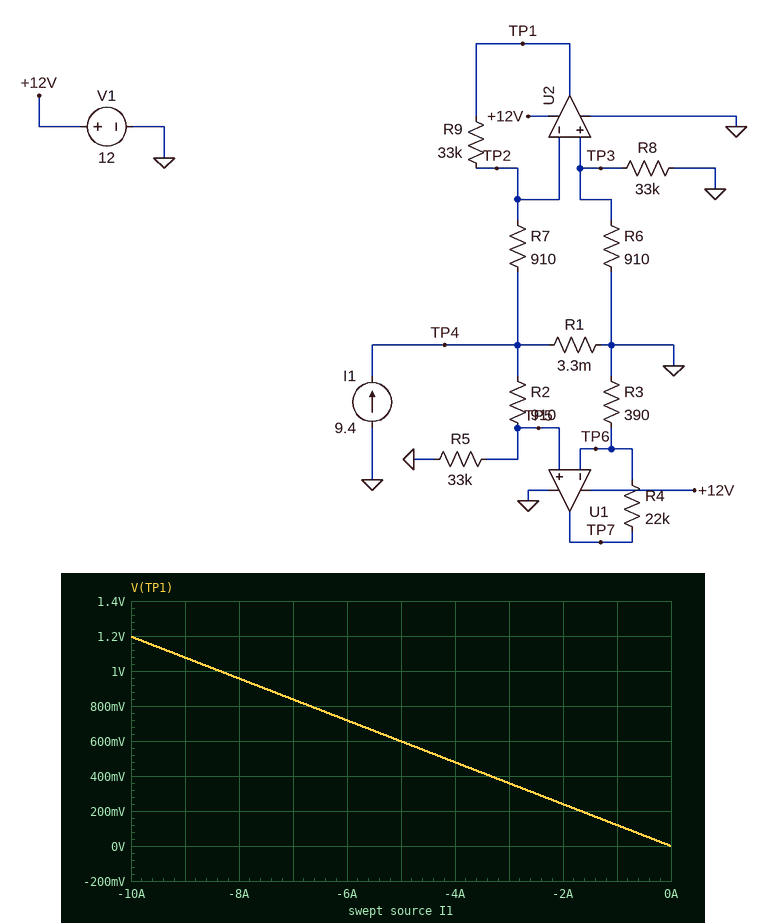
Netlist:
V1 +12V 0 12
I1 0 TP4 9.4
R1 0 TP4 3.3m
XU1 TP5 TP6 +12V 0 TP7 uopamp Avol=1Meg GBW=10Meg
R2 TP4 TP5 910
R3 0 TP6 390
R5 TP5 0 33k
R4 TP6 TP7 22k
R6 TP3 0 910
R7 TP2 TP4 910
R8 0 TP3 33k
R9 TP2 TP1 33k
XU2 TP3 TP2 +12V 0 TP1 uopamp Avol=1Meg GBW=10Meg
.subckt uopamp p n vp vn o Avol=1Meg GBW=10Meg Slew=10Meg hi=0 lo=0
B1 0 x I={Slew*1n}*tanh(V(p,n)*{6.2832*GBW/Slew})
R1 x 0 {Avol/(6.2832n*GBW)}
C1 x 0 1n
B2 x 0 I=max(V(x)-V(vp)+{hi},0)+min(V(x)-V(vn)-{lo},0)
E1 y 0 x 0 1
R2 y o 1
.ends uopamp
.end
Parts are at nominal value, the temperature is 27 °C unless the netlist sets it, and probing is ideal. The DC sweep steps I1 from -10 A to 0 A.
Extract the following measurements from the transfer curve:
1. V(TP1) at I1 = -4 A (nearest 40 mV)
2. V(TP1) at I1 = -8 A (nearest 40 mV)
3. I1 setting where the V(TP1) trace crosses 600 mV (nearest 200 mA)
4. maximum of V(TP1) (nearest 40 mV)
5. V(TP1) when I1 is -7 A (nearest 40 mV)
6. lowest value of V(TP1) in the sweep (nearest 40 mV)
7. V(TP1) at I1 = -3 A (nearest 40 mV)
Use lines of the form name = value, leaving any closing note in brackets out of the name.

V(TP1) at I1 = -4 A = 480 mV
V(TP1) at I1 = -8 A = 960 mV
I1 setting where the V(TP1) trace crosses 600 mV = -5.0 A
maximum of V(TP1) = 1.20 V
V(TP1) when I1 is -7 A = 840 mV
lowest value of V(TP1) in the sweep = 0 V
V(TP1) at I1 = -3 A = 360 mV
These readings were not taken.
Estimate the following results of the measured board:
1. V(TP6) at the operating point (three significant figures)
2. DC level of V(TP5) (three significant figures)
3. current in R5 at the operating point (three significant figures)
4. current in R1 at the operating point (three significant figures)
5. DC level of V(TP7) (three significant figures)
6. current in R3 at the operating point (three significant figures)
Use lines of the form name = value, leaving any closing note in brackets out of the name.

V(TP6) at the operating point = 30.2 mV
DC level of V(TP5) = 30.2 mV
current in R5 at the operating point = 915 nA
current in R1 at the operating point = 9.40 A
DC level of V(TP7) = 1.73 V
current in R3 at the operating point = 77.4 µA
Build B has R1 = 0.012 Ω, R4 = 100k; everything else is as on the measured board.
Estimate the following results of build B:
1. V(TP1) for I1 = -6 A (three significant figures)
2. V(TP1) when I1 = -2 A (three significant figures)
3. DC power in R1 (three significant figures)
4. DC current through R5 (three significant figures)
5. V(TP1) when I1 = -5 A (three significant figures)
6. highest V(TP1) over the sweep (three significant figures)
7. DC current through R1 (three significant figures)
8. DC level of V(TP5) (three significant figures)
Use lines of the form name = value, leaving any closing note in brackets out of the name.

V(TP1) for I1 = -6 A = 2.61 V
V(TP1) when I1 = -2 A = 870 mV
DC power in R1 = 1.06 W
DC current through R5 = 3.33 µA
V(TP1) when I1 = -5 A = 2.18 V
highest V(TP1) over the sweep = 4.35 V
DC current through R1 = 9.40 A
DC level of V(TP5) = 110 mV
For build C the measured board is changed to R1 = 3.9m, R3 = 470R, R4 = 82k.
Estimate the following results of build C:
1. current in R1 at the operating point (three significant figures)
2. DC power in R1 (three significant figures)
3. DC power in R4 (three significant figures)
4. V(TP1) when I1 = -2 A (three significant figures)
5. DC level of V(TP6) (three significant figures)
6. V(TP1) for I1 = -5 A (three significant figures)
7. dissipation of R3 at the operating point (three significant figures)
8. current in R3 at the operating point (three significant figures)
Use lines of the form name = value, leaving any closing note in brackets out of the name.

current in R1 at the operating point = 9.40 A
DC power in R1 = 345 mW
DC power in R4 = 472 µW
V(TP1) when I1 = -2 A = 283 mV
DC level of V(TP6) = 35.7 mV
V(TP1) for I1 = -5 A = 707 mV
dissipation of R3 at the operating point = 2.71 µW
current in R3 at the operating point = 75.9 µA
